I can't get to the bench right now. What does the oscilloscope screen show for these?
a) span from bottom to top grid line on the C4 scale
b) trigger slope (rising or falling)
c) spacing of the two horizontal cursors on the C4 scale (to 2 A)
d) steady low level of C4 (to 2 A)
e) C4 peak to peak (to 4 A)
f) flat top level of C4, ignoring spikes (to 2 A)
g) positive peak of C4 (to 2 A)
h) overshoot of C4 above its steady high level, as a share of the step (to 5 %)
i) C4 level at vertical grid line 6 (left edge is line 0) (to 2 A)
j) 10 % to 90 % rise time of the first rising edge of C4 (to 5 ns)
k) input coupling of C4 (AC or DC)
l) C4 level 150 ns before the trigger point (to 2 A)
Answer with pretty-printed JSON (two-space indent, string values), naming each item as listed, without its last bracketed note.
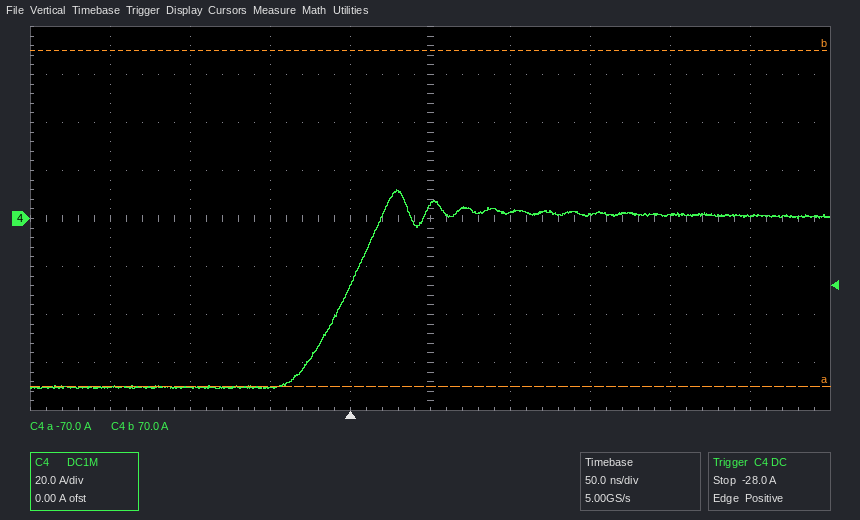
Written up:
{
  "span from bottom to top grid line on the C4 scale": "160 A",
  "trigger slope": "rising",
  "spacing of the two horizontal cursors on the C4 scale": "140 A",
  "steady low level of C4": "-70 A",
  "C4 peak to peak": "84 A",
  "flat top level of C4, ignoring spikes": "2 A",
  "positive peak of C4": "12 A",
  "overshoot of C4 above its steady high level, as a share of the step": "15 %",
  "C4 level at vertical grid line 6 (left edge is line 0)": "2 A",
  "10 % to 90 % rise time of the first rising edge of C4": "45 ns",
  "input coupling of C4": "DC",
  "C4 level 150 ns before the trigger point": "-70 A"
}
